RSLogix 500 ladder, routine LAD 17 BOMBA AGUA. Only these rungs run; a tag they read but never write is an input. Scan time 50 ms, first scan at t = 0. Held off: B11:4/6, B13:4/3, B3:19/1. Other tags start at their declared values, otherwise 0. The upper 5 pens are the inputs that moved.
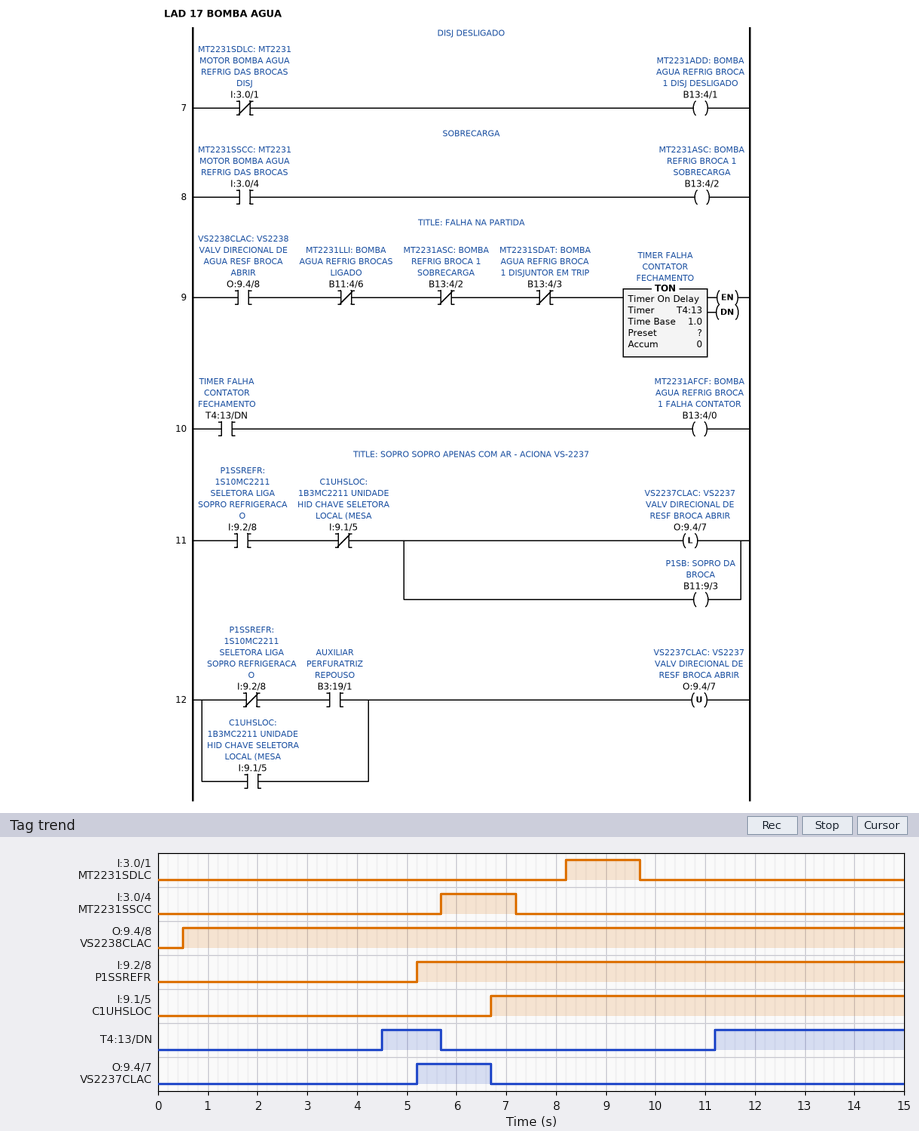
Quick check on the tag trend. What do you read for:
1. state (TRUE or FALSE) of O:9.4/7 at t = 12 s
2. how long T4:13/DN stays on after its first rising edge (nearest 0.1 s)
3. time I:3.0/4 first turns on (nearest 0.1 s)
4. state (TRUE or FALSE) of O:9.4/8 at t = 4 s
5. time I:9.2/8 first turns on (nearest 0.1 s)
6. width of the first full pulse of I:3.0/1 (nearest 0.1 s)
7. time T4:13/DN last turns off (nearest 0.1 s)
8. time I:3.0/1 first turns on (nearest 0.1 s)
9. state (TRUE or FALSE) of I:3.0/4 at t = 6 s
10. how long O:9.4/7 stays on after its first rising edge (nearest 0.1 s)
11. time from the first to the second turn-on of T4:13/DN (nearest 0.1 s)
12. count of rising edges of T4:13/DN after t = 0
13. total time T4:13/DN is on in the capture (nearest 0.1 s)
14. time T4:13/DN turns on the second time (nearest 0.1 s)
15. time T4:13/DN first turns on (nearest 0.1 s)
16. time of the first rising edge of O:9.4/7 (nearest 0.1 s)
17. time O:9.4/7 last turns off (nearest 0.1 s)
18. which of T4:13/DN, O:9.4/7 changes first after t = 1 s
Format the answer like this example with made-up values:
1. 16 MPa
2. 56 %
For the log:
1. FALSE
2. 1.2 s
3. 5.7 s
4. TRUE
5. 5.2 s
6. 1.5 s
7. 5.7 s
8. 8.2 s
9. TRUE
10. 1.5 s
11. 6.7 s
12. 2
13. 5.0 s
14. 11.2 s
15. 4.5 s
16. 5.2 s
17. 6.7 s
18. T4:13/DN
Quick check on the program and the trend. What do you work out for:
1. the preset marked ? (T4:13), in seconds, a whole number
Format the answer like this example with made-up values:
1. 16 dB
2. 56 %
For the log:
1. 4 s
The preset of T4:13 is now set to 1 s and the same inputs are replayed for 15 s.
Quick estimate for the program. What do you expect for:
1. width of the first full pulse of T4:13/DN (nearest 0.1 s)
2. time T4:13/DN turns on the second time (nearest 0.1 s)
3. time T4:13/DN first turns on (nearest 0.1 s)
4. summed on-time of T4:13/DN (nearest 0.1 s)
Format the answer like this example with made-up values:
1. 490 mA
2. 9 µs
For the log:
1. 4.2 s
2. 8.2 s
3. 1.5 s
4. 11.0 s
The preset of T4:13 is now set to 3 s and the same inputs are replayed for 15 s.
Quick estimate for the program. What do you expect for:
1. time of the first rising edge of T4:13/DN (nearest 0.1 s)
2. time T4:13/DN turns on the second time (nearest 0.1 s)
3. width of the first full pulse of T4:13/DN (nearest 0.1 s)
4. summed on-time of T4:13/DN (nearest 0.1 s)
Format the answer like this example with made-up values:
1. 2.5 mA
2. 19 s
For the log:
1. 3.5 s
2. 10.2 s
3. 2.2 s
4. 7.0 s
